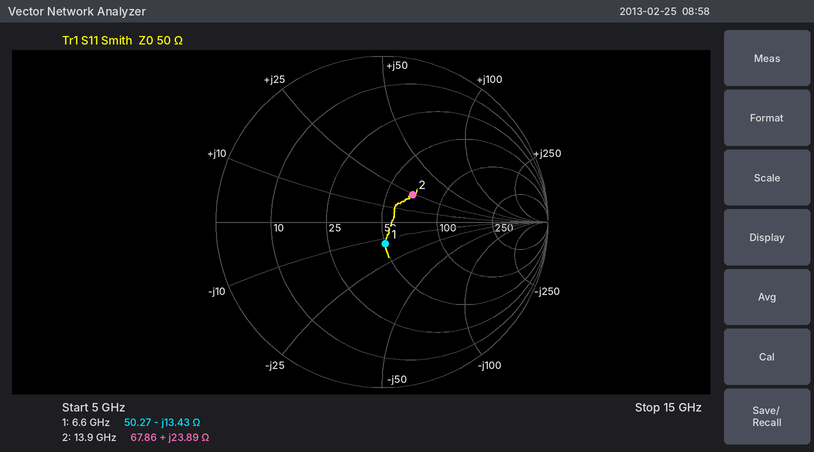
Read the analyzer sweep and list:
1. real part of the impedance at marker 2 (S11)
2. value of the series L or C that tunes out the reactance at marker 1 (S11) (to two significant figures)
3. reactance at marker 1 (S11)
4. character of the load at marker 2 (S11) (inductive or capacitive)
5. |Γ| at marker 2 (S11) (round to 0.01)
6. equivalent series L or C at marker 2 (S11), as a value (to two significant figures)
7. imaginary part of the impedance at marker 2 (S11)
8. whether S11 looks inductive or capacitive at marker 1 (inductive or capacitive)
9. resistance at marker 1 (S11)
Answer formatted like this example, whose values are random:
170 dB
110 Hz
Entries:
67.86 Ω
320 pH
-13.43 Ω
inductive
0.25
270 pH
+23.89 Ω
capacitive
50.27 Ω
